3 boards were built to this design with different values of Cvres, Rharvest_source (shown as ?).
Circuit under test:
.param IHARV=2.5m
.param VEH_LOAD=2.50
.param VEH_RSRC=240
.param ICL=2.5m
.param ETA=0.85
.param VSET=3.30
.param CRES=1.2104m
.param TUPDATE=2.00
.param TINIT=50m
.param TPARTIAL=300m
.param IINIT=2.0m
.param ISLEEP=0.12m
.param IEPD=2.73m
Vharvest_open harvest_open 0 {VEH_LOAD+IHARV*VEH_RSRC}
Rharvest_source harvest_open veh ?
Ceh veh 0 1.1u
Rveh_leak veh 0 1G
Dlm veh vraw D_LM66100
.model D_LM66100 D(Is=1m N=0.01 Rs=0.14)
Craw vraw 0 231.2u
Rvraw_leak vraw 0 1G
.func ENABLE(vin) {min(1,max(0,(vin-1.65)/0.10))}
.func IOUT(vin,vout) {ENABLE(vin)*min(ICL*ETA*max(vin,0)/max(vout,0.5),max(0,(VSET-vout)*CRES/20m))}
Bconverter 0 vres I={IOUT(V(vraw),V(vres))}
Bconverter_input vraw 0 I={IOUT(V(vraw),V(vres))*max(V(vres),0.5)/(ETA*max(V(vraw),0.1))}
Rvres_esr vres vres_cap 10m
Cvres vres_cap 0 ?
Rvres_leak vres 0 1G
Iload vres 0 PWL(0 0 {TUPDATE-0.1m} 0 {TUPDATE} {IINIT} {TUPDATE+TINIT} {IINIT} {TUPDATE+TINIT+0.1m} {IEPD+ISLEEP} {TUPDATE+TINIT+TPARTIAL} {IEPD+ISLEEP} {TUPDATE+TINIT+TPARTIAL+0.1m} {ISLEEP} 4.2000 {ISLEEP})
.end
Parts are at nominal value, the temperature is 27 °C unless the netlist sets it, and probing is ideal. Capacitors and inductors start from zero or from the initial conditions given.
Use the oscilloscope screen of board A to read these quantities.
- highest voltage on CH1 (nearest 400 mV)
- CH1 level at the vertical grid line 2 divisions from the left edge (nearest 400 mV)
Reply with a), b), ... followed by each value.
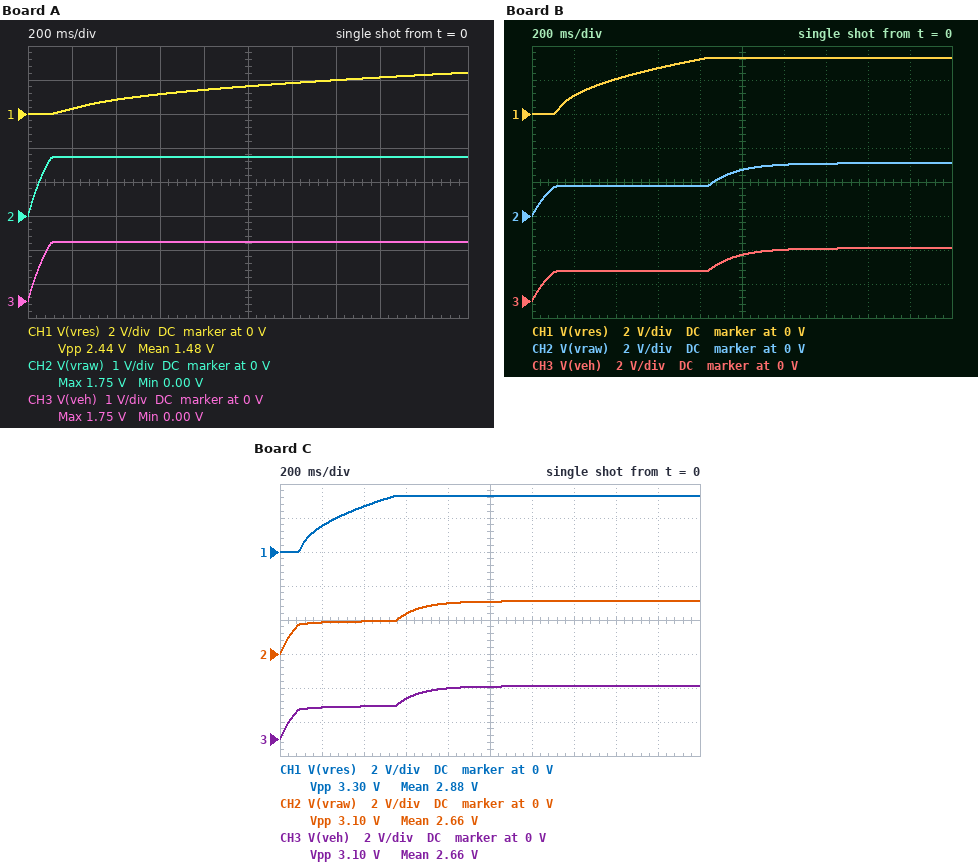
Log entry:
a) 2.4 V
b) 800 mV
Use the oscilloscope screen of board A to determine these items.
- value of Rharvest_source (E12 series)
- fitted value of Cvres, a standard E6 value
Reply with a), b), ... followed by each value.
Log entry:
a) 560 Ω
b) 2.2 mF
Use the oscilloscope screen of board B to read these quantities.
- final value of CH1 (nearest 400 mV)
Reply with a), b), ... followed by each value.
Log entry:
a) 3.2 V
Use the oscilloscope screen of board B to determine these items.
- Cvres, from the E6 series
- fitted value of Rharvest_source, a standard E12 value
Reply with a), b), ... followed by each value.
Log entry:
a) 470 µF
b) 560 Ω
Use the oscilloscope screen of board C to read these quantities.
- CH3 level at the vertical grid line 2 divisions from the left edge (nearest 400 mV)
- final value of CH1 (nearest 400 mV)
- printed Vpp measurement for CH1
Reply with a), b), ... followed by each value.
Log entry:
a) 2.0 V
b) 3.2 V
c) 3.30 V
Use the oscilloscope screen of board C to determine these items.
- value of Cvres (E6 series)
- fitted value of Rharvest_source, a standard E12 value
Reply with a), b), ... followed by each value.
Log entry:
a) 330 µF
b) 470 Ω
